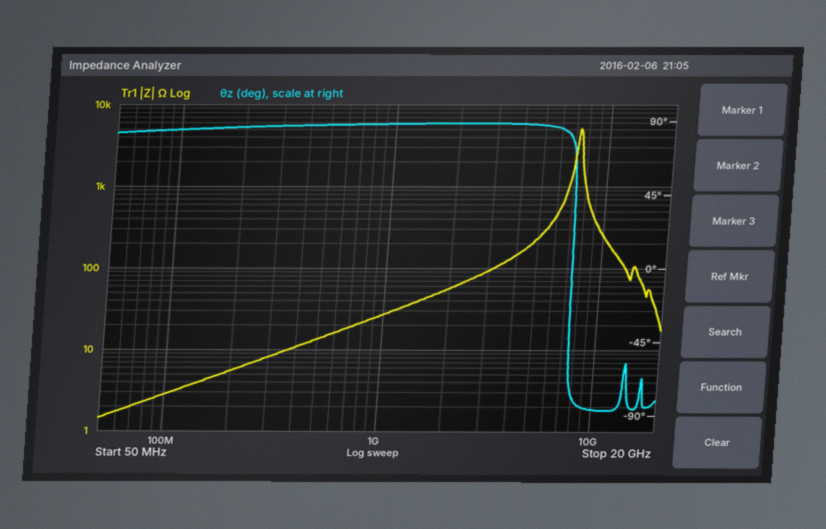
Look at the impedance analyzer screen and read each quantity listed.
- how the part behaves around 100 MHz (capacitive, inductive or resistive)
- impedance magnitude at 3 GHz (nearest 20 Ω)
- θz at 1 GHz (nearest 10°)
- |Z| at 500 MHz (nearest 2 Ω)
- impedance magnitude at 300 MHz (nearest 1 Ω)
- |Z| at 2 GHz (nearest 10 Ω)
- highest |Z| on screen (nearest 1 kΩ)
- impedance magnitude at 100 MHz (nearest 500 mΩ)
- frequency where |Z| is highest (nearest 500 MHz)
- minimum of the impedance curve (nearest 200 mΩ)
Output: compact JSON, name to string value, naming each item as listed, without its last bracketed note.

{"how the part behaves around 100 MHz": "inductive", "impedance magnitude at 3 GHz": "100 Ω", "θz at 1 GHz": "90°", "|Z| at 500 MHz": "14 Ω", "impedance magnitude at 300 MHz": "8 Ω", "|Z| at 2 GHz": "60 Ω", "highest |Z| on screen": "5 kΩ", "impedance magnitude at 100 MHz": "3.0 Ω", "frequency where |Z| is highest": "7.5 GHz", "minimum of the impedance curve": "1.4 Ω"}
